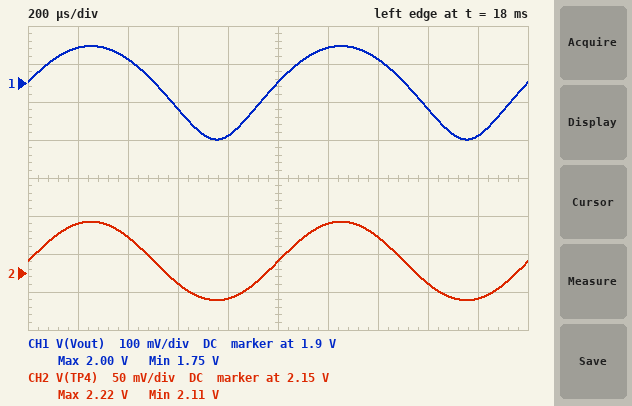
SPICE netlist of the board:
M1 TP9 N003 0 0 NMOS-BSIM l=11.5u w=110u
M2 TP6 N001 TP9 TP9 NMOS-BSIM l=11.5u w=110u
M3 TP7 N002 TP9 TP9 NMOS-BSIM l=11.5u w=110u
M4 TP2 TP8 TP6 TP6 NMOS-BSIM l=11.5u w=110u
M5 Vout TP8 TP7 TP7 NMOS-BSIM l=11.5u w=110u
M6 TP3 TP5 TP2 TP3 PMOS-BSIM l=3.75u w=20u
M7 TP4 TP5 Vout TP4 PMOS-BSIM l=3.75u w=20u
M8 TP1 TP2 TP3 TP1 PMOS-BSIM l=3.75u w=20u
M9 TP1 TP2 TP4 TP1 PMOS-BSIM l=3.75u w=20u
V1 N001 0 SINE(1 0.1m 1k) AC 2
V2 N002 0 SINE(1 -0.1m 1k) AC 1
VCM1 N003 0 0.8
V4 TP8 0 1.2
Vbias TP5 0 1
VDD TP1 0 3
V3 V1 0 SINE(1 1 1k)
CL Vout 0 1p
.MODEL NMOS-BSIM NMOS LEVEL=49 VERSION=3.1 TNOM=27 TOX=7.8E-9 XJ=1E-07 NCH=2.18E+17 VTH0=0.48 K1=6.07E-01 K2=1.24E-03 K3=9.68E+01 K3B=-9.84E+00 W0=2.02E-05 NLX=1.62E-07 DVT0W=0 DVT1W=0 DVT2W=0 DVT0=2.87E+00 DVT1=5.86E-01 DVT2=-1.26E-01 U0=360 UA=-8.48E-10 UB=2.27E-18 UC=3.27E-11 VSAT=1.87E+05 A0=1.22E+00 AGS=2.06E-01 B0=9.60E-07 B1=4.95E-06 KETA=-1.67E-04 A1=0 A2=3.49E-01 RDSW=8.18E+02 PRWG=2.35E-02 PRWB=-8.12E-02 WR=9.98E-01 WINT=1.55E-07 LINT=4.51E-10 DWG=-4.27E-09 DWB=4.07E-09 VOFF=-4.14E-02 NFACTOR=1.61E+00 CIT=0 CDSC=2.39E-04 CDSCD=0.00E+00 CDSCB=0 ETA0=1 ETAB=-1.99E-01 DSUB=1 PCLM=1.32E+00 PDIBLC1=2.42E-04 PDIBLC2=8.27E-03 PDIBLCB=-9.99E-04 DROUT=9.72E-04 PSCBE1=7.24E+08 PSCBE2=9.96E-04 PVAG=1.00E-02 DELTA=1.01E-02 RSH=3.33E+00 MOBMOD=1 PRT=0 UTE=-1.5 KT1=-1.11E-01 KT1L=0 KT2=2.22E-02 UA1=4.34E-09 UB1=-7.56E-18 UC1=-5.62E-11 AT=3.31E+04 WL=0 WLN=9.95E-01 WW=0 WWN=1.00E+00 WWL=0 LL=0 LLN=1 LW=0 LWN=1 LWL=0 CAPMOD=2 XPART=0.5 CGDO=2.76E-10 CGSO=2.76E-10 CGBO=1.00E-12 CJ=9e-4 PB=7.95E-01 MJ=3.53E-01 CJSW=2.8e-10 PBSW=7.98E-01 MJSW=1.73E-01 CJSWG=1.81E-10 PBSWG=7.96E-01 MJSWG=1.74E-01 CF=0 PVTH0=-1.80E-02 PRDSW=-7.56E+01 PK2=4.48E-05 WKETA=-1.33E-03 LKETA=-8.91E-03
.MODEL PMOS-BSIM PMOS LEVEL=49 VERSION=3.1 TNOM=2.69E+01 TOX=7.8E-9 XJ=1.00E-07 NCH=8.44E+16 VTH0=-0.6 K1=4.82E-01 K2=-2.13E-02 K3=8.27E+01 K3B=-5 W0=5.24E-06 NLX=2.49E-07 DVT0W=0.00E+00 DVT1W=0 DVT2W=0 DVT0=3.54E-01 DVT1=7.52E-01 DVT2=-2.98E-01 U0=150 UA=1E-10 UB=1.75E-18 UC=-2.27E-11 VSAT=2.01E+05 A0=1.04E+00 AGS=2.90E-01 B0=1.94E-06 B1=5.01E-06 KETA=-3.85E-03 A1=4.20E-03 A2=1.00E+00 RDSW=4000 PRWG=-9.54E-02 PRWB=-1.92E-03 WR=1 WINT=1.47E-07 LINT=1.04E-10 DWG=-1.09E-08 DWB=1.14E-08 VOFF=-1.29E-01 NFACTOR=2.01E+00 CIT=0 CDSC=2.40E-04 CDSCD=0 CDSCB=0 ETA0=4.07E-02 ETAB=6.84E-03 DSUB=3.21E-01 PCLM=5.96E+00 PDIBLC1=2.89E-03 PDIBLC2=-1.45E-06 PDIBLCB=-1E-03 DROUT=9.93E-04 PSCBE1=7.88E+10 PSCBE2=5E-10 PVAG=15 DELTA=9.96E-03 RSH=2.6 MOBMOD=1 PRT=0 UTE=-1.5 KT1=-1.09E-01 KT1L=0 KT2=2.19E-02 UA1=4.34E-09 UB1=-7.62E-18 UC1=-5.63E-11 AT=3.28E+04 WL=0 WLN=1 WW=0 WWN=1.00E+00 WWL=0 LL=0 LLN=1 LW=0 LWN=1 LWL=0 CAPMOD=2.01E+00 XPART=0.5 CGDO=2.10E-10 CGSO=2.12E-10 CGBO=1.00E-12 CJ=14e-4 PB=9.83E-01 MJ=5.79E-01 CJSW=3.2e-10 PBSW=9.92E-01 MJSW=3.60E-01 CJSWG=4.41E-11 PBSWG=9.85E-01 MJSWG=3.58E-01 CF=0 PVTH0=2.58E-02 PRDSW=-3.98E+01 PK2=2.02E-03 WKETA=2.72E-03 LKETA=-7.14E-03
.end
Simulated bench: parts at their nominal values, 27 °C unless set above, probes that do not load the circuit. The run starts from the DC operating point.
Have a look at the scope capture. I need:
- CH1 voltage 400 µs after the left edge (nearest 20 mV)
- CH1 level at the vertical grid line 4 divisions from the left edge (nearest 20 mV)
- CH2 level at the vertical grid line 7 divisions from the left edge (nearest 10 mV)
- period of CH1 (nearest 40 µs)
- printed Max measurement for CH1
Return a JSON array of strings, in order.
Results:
["1.96 V", "1.76 V", "2.20 V", "1.00 ms", "2.00 V"]
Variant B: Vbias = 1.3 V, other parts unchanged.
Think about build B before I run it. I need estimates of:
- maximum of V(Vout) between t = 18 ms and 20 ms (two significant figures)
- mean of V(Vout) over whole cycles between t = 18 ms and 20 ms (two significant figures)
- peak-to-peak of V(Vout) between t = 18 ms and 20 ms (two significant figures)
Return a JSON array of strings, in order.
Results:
["2.1 V", "1.7 V", "1.1 V"]
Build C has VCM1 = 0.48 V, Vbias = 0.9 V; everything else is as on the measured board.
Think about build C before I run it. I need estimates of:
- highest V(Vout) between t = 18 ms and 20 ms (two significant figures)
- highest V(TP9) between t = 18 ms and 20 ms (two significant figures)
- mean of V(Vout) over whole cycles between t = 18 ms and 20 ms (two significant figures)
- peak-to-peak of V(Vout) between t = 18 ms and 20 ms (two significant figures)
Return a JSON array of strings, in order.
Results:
["2.5 V", "550 mV", "2.4 V", "150 mV"]
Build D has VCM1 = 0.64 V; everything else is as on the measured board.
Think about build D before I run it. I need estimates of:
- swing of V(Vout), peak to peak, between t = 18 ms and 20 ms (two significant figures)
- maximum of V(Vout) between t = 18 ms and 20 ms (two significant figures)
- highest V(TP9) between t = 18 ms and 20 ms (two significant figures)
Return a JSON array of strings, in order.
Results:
["220 mV", "2.3 V", "400 mV"]
